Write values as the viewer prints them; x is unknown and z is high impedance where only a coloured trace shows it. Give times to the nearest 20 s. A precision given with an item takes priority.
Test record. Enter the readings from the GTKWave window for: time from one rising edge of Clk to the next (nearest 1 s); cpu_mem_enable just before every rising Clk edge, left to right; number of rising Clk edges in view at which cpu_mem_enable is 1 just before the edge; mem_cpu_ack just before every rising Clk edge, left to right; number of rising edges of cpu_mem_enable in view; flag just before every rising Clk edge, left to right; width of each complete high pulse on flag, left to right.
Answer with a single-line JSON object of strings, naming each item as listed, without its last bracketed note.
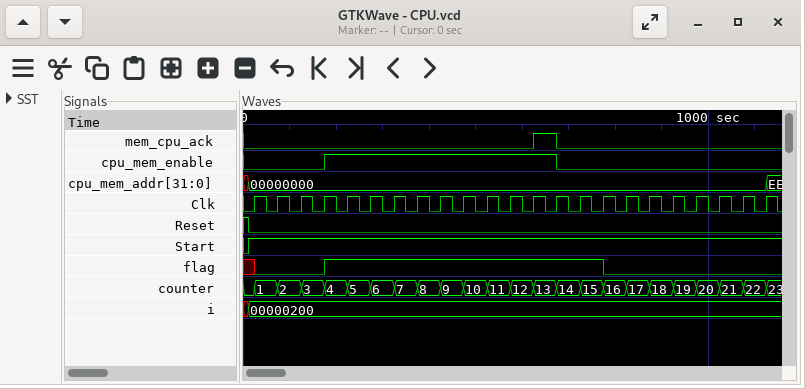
{"time from one rising edge of Clk to the next": "50 s", "cpu_mem_enable just before every rising Clk edge, left to right": "0 0 0 0 1 1 1 1 1 1 1 1 1 1 0 0 0 0 0 0 0 0 0", "number of rising Clk edges in view at which cpu_mem_enable is 1 just before the edge": "10", "mem_cpu_ack just before every rising Clk edge, left to right": "0 0 0 0 0 0 0 0 0 0 0 0 0 1 0 0 0 0 0 0 0 0 0", "number of rising edges of cpu_mem_enable in view": "1", "flag just before every rising Clk edge, left to right": "x 0 0 0 1 1 1 1 1 1 1 1 1 1 1 1 0 0 0 0 0 0 0", "width of each complete high pulse on flag, left to right": "600 s"}
